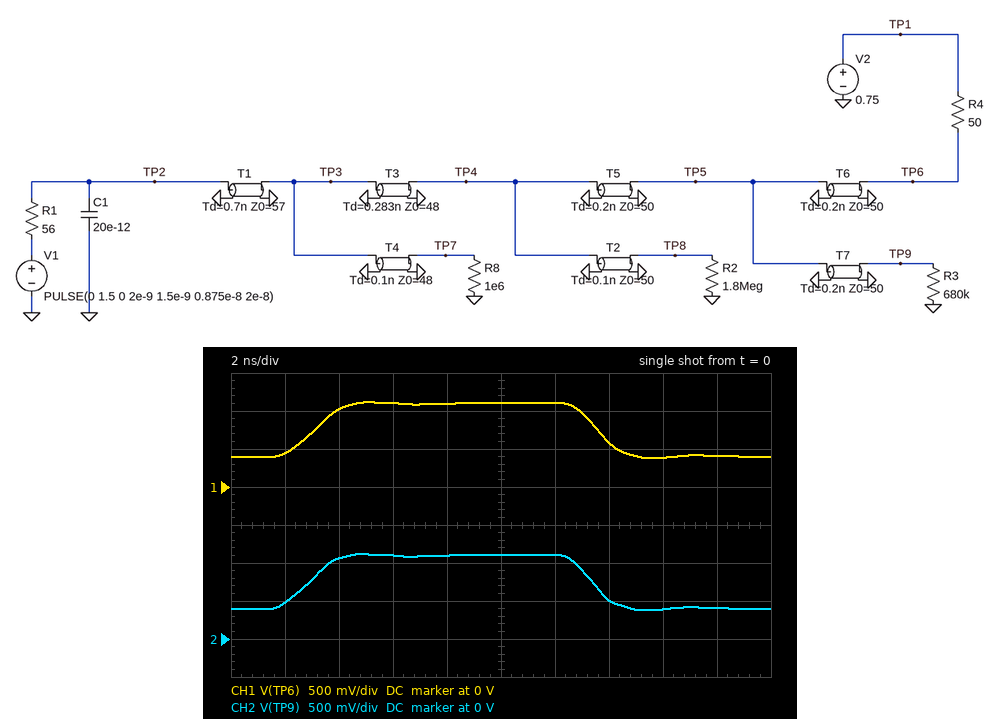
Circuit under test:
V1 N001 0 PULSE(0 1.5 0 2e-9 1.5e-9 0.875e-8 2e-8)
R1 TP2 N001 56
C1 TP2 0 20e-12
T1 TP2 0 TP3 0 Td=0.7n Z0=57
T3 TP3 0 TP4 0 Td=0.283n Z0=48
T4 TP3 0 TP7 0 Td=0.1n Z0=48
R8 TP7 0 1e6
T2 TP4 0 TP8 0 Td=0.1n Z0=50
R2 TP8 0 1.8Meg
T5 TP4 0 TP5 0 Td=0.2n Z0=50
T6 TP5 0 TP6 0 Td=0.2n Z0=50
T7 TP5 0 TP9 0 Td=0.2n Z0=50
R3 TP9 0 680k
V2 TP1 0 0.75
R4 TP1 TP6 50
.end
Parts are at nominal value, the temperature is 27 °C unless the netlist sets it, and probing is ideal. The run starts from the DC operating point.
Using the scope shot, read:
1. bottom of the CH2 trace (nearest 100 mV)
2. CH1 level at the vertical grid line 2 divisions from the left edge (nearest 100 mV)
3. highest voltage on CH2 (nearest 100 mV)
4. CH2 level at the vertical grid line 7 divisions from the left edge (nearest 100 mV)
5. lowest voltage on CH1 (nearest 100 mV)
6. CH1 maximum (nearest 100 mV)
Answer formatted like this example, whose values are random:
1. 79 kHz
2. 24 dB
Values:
1. 400 mV
2. 1.0 V
3. 1.1 V
4. 500 mV
5. 400 mV
6. 1.1 V
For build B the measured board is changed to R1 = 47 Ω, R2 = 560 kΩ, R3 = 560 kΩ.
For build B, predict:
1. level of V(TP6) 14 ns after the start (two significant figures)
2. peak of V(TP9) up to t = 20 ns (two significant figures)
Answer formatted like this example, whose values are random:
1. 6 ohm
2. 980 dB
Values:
1. 550 mV
2. 1.2 V
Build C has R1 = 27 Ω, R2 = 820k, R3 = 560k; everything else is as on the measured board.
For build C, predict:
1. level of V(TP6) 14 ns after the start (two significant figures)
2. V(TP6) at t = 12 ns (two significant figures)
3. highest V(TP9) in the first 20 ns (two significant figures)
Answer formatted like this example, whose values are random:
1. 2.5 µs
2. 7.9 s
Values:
1. 430 mV
2. 1.2 V
3. 1.3 V
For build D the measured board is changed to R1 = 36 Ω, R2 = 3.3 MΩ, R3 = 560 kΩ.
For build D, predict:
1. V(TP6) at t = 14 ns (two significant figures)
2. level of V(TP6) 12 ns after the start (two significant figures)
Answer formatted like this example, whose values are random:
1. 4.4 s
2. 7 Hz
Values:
1. 500 mV
2. 1.2 V
